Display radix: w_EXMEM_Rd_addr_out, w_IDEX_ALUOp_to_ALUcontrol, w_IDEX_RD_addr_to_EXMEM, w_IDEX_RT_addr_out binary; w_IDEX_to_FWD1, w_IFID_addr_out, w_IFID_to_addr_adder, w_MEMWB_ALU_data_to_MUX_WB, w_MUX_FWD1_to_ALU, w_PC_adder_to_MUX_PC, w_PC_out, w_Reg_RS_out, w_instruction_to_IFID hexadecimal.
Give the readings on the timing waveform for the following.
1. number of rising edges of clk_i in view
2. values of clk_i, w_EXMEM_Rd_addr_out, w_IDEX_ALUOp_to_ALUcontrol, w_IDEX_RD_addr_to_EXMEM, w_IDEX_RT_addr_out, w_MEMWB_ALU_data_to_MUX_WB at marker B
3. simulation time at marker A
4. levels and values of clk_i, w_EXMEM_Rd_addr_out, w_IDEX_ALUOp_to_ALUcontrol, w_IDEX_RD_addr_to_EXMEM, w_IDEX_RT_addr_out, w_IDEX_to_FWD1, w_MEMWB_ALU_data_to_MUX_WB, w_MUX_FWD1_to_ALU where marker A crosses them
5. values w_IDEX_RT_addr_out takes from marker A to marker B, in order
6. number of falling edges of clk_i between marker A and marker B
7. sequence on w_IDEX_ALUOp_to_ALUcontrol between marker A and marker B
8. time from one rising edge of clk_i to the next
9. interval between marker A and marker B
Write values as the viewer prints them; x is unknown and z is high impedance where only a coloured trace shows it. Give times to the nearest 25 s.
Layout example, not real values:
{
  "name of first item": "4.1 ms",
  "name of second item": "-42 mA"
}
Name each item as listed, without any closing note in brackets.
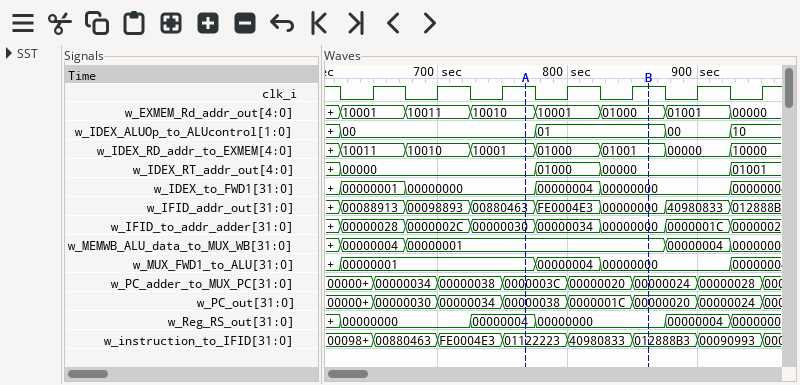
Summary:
{
  "number of rising edges of clk_i in view": "7",
  "values of clk_i, w_EXMEM_Rd_addr_out, w_IDEX_ALUOp_to_ALUcontrol, w_IDEX_RD_addr_to_EXMEM, w_IDEX_RT_addr_out, w_MEMWB_ALU_data_to_MUX_WB at marker B": "clk_i=1, w_EXMEM_Rd_addr_out=01000, w_IDEX_ALUOp_to_ALUcontrol=01, w_IDEX_RD_addr_to_EXMEM=01001, w_IDEX_RT_addr_out=00000, w_MEMWB_ALU_data_to_MUX_WB=00000001",
  "simulation time at marker A": "775 s",
  "levels and values of clk_i, w_EXMEM_Rd_addr_out, w_IDEX_ALUOp_to_ALUcontrol, w_IDEX_RD_addr_to_EXMEM, w_IDEX_RT_addr_out, w_IDEX_to_FWD1, w_MEMWB_ALU_data_to_MUX_WB, w_MUX_FWD1_to_ALU where marker A crosses them": "clk_i=1, w_EXMEM_Rd_addr_out=10010, w_IDEX_ALUOp_to_ALUcontrol=00, w_IDEX_RD_addr_to_EXMEM=10001, w_IDEX_RT_addr_out=00000, w_IDEX_to_FWD1=00000000, w_MEMWB_ALU_data_to_MUX_WB=00000001, w_MUX_FWD1_to_ALU=00000001",
  "values w_IDEX_RT_addr_out takes from marker A to marker B, in order": "00000, 01000, 00000",
  "number of falling edges of clk_i between marker A and marker B": "2",
  "sequence on w_IDEX_ALUOp_to_ALUcontrol between marker A and marker B": "00, 01",
  "time from one rising edge of clk_i to the next": "50 s",
  "interval between marker A and marker B": "100 s"
}
